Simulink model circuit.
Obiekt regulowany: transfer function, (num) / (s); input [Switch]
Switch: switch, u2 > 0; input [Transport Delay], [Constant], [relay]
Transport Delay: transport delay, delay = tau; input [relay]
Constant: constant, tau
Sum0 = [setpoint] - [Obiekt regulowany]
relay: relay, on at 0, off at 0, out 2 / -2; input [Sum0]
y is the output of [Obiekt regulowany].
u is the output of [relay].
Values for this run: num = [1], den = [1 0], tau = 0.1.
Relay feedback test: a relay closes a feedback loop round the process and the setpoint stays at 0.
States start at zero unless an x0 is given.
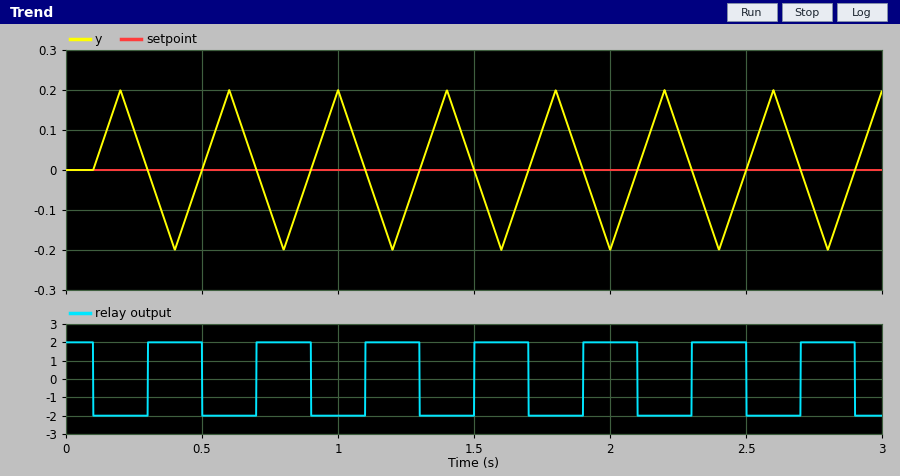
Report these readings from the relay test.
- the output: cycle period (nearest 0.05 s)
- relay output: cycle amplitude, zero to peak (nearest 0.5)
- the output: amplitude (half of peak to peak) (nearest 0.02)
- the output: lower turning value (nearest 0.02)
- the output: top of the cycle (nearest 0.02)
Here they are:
0.40 s
2.0
0.20
-0.20
0.20
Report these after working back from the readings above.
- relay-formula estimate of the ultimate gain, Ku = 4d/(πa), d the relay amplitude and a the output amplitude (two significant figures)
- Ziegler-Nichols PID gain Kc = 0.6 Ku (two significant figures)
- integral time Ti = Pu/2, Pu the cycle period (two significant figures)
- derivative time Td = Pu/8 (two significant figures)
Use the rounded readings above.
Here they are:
13
7.8
0.20 s
0.050 s
